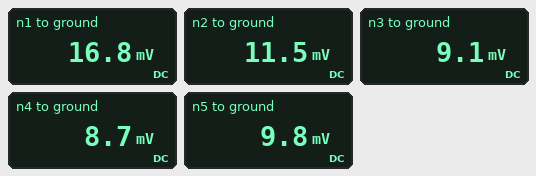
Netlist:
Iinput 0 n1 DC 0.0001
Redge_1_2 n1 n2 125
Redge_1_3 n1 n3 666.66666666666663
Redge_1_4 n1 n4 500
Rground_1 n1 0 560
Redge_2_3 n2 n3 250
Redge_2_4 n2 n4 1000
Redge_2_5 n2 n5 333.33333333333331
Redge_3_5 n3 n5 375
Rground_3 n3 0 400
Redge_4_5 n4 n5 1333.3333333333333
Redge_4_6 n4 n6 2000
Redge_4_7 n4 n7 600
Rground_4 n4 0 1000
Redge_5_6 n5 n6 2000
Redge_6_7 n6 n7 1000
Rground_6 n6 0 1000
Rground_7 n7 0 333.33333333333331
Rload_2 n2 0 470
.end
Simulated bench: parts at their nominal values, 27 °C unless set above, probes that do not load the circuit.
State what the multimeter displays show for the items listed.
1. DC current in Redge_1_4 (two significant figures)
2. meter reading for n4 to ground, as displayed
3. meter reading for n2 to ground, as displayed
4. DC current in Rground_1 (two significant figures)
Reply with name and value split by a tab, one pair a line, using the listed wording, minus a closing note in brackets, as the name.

DC current in Redge_1_4	16 µA
meter reading for n4 to ground, as displayed	8.7 mV
meter reading for n2 to ground, as displayed	11.5 mV
DC current in Rground_1	30 µA
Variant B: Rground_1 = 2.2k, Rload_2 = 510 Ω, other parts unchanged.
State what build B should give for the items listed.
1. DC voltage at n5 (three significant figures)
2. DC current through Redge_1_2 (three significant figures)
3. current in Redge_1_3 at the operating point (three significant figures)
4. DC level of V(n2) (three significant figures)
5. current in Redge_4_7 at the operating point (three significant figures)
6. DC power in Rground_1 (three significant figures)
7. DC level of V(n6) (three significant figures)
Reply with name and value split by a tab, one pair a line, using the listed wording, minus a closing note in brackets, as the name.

DC voltage at n5	12.9 mV
DC current through Redge_1_2	53.9 µA
current in Redge_1_3 at the operating point	14.9 µA
DC level of V(n2)	15.3 mV
current in Redge_4_7 at the operating point	11.8 µA
DC power in Rground_1	220 nW
DC level of V(n6)	5.50 mV
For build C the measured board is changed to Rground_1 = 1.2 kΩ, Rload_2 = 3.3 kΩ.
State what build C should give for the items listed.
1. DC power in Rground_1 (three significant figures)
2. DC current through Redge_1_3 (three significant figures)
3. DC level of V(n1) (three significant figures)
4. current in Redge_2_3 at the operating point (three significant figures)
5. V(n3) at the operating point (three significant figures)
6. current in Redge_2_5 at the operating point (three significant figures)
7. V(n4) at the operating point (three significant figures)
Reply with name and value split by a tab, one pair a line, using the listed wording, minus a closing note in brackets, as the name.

DC power in Rground_1	518 nW
DC current through Redge_1_3	14.9 µA
DC level of V(n1)	24.9 mV
current in Redge_2_3 at the operating point	19.0 µA
V(n3) at the operating point	15.0 mV
current in Redge_2_5 at the operating point	10.3 µA
V(n4) at the operating point	13.6 mV
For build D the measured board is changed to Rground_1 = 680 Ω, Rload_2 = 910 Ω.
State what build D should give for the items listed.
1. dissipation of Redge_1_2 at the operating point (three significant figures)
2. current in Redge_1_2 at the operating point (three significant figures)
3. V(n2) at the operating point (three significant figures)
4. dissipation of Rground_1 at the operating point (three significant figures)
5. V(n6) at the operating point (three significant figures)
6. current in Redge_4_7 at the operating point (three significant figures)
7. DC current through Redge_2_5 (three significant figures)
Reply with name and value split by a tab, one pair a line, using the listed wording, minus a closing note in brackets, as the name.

dissipation of Redge_1_2 at the operating point	204 nW
current in Redge_1_2 at the operating point	40.4 µA
V(n2) at the operating point	14.5 mV
dissipation of Rground_1 at the operating point	562 nW
V(n6) at the operating point	5.06 mV
current in Redge_4_7 at the operating point	10.7 µA
DC current through Redge_2_5	7.19 µA
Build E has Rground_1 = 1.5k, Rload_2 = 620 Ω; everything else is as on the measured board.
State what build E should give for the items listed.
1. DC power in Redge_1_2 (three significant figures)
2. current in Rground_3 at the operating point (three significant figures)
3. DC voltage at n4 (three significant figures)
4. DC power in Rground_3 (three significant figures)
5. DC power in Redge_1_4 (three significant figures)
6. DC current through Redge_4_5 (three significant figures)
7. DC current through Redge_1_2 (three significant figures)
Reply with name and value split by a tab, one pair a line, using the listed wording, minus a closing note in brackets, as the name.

DC power in Redge_1_2	315 nW
current in Rground_3 at the operating point	30.4 µA
DC voltage at n4	11.4 mV
DC power in Rground_3	370 nW
DC power in Redge_1_4	216 nW
DC current through Redge_4_5	1.24 µA
DC current through Redge_1_2	50.2 µA
